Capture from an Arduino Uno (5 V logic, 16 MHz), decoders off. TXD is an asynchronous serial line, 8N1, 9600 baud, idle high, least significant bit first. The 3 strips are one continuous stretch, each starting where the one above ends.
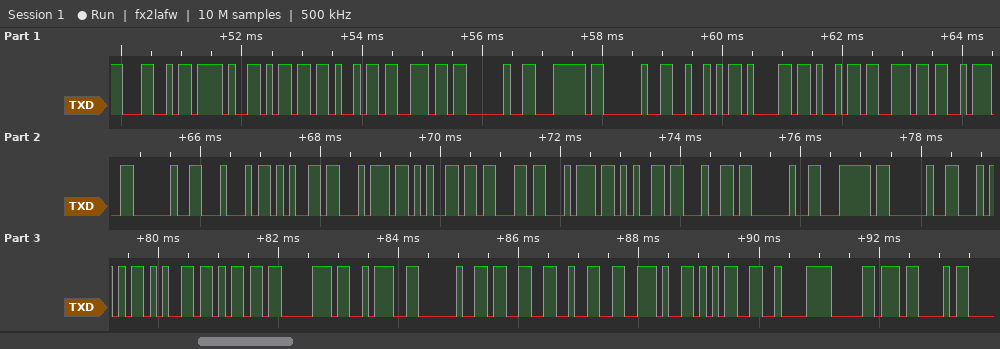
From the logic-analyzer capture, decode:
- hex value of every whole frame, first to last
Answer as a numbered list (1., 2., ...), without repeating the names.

1. 0x4C 0x2F 0x6D 0x69 0x6E 0x20 0x7C 0x20 0x52 0x61 0x69 0x6E 0x3A 0x20 0x44 0x65 0x74 0x65 0x63 0x74 0x65 0x64 0x20 0x7C 0x20 0x54 0x65 0x6D 0x70 0x3A 0x20 0x33 0x32 0x2E 0x35 0xC2 0xB0 0x43
